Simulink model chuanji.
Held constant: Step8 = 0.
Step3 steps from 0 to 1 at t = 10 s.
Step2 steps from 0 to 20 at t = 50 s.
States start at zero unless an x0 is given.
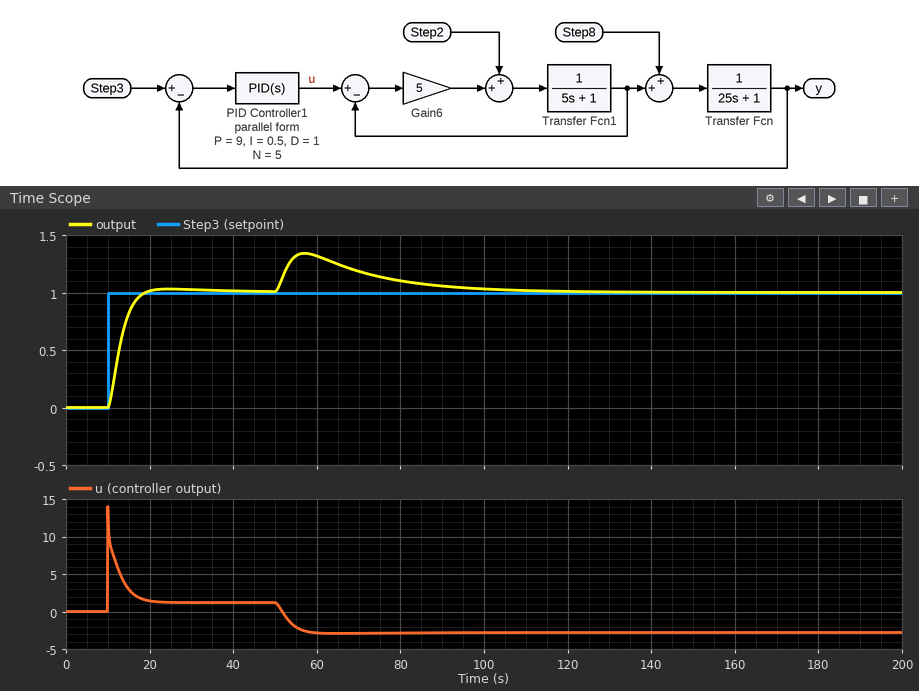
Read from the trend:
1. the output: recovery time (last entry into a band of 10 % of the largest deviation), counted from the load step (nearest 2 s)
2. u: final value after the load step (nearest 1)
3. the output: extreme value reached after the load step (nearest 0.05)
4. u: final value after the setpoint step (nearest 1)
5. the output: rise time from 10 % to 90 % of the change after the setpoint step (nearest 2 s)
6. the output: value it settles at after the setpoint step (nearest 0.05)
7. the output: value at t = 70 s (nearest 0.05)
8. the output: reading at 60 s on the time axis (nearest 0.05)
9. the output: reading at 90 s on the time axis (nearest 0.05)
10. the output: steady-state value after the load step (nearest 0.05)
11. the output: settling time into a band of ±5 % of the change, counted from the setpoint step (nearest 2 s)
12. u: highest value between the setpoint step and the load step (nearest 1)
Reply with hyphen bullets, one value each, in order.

- 48 s
- -3
- 1.35
- 1
- 6 s
- 1.00
- 1.20
- 1.30
- 1.05
- 1.00
- 8 s
- 14
